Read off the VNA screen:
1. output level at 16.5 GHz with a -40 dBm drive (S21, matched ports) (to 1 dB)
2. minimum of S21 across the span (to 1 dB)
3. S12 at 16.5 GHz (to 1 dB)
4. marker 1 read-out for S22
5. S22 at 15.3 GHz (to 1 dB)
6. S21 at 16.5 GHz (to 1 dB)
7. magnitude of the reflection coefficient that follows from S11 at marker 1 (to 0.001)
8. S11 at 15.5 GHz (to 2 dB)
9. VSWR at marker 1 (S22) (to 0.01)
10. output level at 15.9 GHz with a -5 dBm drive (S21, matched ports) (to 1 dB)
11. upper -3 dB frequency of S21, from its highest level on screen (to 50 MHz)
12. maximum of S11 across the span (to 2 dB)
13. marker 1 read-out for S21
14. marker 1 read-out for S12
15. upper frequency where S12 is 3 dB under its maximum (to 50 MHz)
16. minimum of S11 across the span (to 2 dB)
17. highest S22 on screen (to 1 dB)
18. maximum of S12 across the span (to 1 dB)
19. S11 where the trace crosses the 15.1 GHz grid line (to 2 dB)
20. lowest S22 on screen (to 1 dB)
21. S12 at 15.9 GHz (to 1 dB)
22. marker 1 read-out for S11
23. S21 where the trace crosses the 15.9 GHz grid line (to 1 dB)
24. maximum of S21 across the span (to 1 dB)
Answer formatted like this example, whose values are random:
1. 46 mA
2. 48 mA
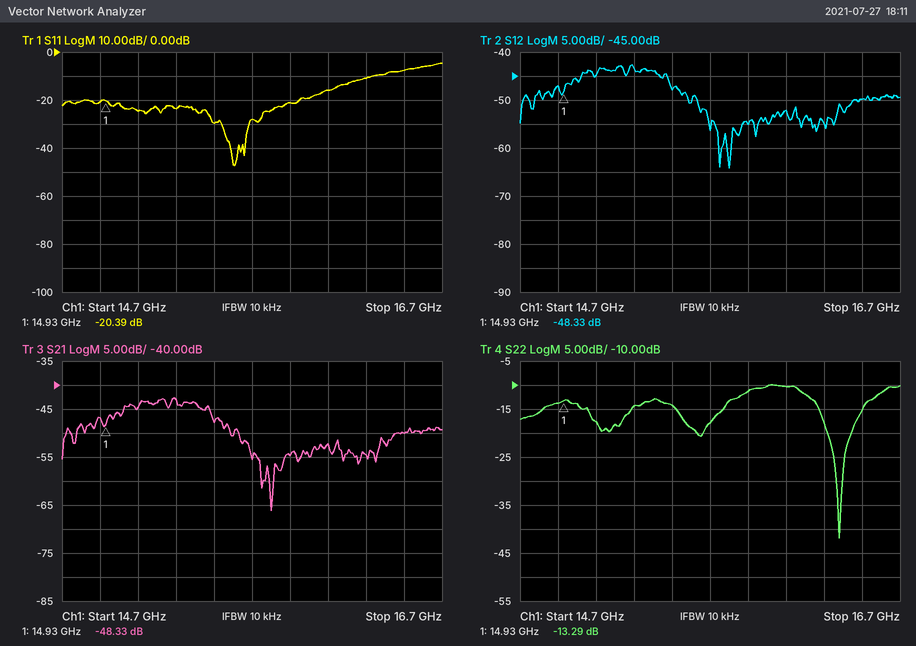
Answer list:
1. -90 dBm
2. -66 dB
3. -50 dB
4. -13.29 dB
5. -14 dB
6. -50 dB
7. 0.096
8. -30 dB
9. 1.55
10. -60 dBm
11. 15.50 GHz
12. -4 dB
13. -48.33 dB
14. -48.33 dB
15. 15.50 GHz
16. -48 dB
17. -10 dB
18. -43 dB
19. -24 dB
20. -42 dB
21. -55 dB
22. -20.39 dB
23. -55 dB
24. -43 dB
